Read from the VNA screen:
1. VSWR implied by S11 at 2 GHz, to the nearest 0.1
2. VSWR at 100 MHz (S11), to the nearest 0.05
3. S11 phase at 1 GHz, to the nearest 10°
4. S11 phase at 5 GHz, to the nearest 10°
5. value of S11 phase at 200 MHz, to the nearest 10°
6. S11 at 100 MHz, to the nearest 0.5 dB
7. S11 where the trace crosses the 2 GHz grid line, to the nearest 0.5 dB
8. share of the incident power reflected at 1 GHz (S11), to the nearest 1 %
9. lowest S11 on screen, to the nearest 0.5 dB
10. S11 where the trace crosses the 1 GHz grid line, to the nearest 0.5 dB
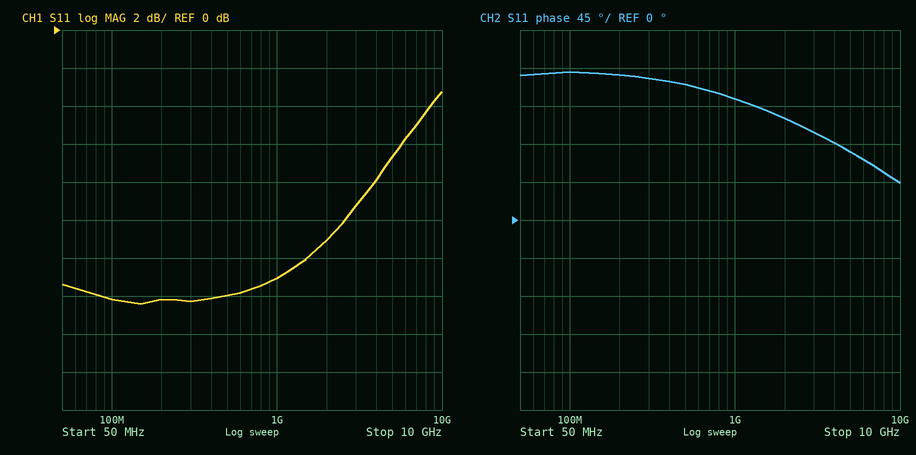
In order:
1.8
1.50
140°
80°
170°
-14.0 dB
-11.0 dB
5 %
-14.5 dB
-13.0 dB
